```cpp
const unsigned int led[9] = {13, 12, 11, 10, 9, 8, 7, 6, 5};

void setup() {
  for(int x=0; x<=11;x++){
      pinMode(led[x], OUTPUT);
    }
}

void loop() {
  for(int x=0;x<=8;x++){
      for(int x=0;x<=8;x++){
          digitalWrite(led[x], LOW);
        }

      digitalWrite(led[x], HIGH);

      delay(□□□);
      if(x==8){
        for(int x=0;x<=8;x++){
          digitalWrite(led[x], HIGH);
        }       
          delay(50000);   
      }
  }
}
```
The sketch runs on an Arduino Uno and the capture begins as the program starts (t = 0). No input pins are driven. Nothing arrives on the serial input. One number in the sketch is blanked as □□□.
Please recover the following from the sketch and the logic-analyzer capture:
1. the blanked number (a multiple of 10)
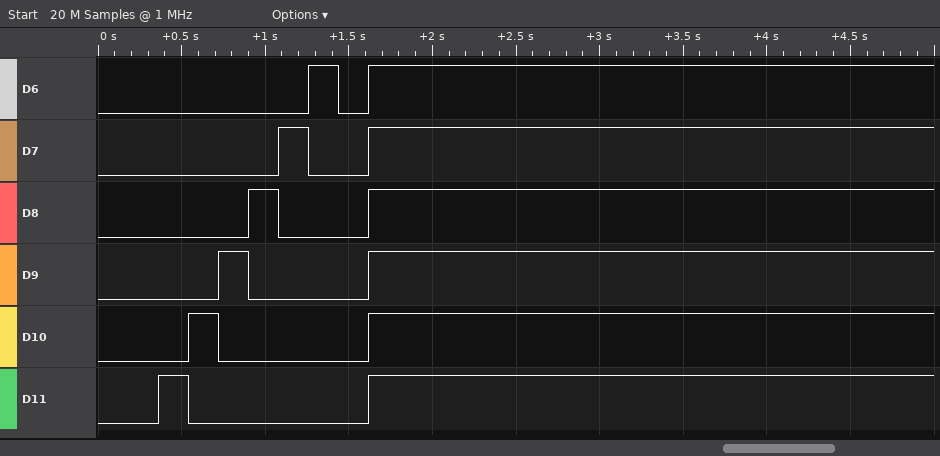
180
